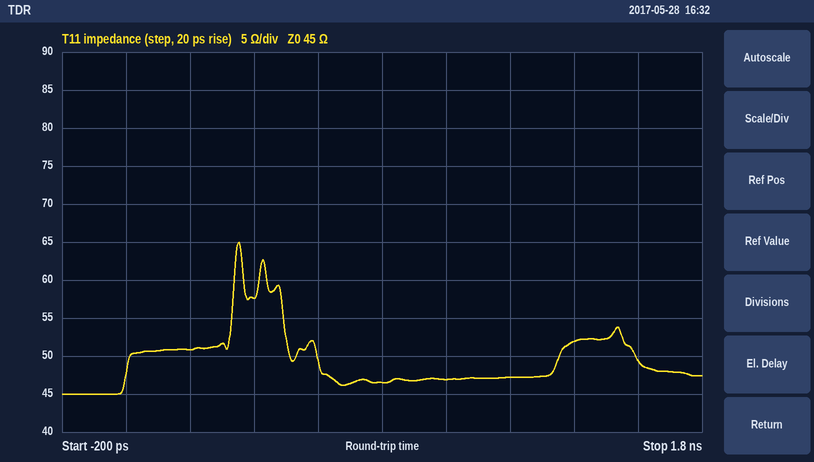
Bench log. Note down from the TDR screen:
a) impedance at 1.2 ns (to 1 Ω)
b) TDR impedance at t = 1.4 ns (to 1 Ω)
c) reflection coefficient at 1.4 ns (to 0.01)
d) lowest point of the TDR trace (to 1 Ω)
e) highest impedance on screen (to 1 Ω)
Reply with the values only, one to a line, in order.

47 Ω
52 Ω
+0.07
45 Ω
65 Ω
